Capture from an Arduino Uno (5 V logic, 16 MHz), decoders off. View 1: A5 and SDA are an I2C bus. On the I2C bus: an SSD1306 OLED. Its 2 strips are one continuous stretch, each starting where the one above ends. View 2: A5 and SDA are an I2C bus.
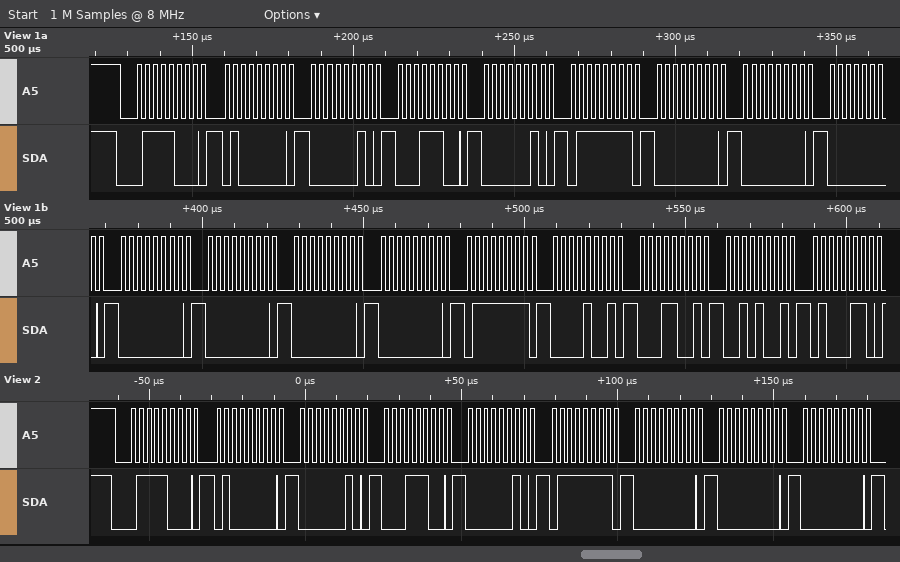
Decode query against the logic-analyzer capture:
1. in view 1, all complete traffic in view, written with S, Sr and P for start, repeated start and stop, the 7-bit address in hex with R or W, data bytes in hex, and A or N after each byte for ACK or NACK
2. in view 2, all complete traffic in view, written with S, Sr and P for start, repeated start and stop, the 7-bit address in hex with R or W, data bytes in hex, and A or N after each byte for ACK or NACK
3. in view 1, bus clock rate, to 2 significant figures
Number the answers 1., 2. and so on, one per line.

1. S 3CW A 40 A 02 A 1C A 02 A 7F A 00 A 00 A 00 A 00 A 00 A 00 A 00 A 7F A 09 A 19 A 29 A 46 A
2. S 3CW A 40 A 02 A 1C A 02 A 7F A 00 A 00 A 00 A
3. 400 kHz
